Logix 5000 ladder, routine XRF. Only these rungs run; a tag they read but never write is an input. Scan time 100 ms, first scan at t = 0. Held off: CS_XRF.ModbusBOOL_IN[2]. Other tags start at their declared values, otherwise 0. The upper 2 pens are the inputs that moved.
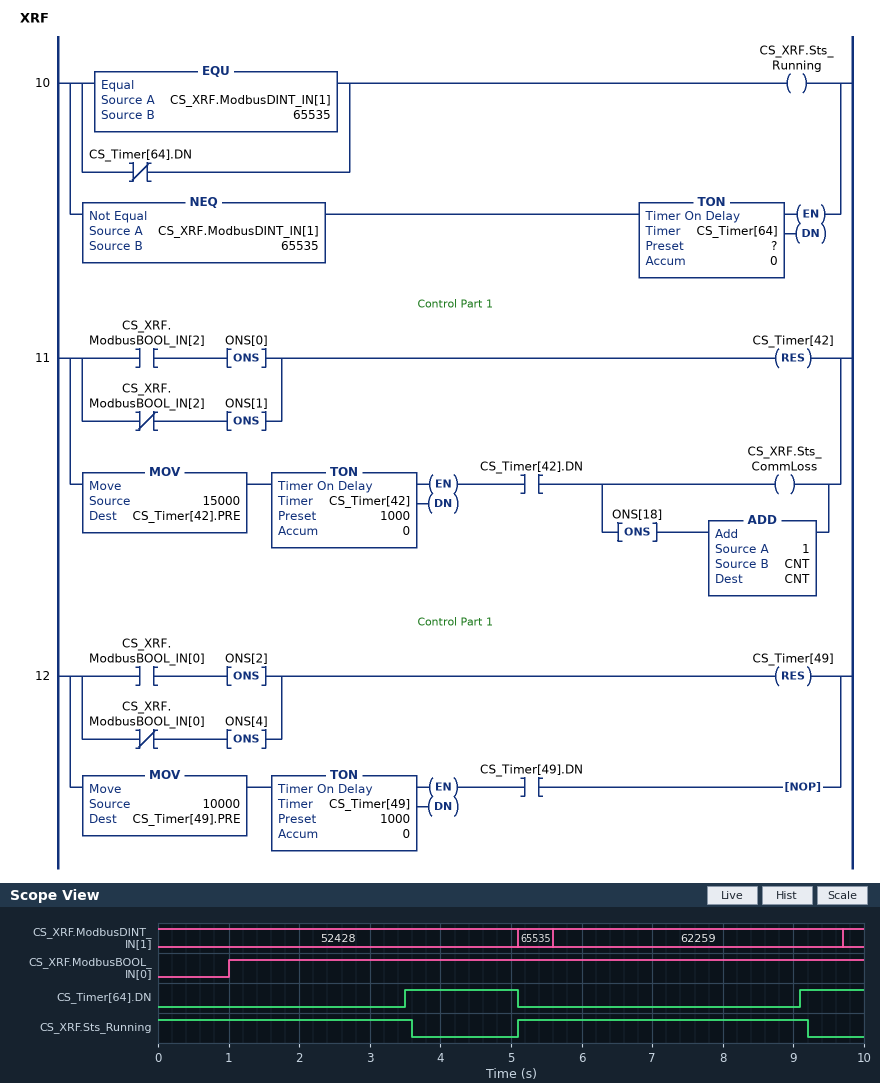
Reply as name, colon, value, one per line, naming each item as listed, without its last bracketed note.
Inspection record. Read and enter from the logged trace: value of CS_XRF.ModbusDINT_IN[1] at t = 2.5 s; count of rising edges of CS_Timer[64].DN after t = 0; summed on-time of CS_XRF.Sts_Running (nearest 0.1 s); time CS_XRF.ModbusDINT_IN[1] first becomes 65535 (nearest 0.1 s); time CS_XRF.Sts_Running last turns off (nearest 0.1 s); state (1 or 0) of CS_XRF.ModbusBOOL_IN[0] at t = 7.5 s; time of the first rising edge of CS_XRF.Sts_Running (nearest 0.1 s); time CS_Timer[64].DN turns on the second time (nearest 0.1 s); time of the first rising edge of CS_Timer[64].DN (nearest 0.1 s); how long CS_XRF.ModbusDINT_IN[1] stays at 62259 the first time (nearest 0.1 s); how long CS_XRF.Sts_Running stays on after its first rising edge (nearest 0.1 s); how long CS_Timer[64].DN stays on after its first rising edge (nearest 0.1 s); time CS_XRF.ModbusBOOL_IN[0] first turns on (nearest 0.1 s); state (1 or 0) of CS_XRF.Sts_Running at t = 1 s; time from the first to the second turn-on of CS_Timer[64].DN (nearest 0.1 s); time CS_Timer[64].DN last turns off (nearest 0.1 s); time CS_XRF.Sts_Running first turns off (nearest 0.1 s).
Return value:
value of CS_XRF.ModbusDINT_IN[1] at t = 2.5 s: 52428
count of rising edges of CS_Timer[64].DN after t = 0: 2
summed on-time of CS_XRF.Sts_Running: 7.7 s
time CS_XRF.ModbusDINT_IN[1] first becomes 65535: 5.1 s
time CS_XRF.Sts_Running last turns off: 9.2 s
state (1 or 0) of CS_XRF.ModbusBOOL_IN[0] at t = 7.5 s: 1
time of the first rising edge of CS_XRF.Sts_Running: 5.1 s
time CS_Timer[64].DN turns on the second time: 9.1 s
time of the first rising edge of CS_Timer[64].DN: 3.5 s
how long CS_XRF.ModbusDINT_IN[1] stays at 62259 the first time: 4.1 s
how long CS_XRF.Sts_Running stays on after its first rising edge: 4.1 s
how long CS_Timer[64].DN stays on after its first rising edge: 1.6 s
time CS_XRF.ModbusBOOL_IN[0] first turns on: 1.0 s
state (1 or 0) of CS_XRF.Sts_Running at t = 1 s: 1
time from the first to the second turn-on of CS_Timer[64].DN: 5.6 s
time CS_Timer[64].DN last turns off: 5.1 s
time CS_XRF.Sts_Running first turns off: 3.6 s
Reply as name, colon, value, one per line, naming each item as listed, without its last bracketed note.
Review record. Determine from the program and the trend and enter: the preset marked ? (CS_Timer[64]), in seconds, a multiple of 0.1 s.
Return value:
the preset marked ? (CS_Timer[64]), in seconds, a multiple of 0.1 s: 3.5 s
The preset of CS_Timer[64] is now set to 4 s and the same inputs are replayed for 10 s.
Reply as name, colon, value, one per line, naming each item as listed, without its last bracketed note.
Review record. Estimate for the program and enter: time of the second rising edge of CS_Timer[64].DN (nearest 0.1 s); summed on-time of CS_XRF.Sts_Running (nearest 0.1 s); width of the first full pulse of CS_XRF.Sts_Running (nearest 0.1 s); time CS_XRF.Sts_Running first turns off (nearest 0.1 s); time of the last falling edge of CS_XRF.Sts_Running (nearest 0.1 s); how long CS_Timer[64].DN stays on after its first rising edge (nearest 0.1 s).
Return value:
time of the second rising edge of CS_Timer[64].DN: 9.6 s
summed on-time of CS_XRF.Sts_Running: 8.7 s
width of the first full pulse of CS_XRF.Sts_Running: 4.6 s
time CS_XRF.Sts_Running first turns off: 4.1 s
time of the last falling edge of CS_XRF.Sts_Running: 9.7 s
how long CS_Timer[64].DN stays on after its first rising edge: 1.1 s
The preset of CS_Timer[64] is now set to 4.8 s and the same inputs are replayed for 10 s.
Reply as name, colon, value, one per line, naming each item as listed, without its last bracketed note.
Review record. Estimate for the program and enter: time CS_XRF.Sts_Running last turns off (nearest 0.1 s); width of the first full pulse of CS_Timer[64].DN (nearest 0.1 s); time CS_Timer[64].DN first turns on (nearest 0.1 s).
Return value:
time CS_XRF.Sts_Running last turns off: 4.9 s
width of the first full pulse of CS_Timer[64].DN: 0.3 s
time CS_Timer[64].DN first turns on: 4.8 s
